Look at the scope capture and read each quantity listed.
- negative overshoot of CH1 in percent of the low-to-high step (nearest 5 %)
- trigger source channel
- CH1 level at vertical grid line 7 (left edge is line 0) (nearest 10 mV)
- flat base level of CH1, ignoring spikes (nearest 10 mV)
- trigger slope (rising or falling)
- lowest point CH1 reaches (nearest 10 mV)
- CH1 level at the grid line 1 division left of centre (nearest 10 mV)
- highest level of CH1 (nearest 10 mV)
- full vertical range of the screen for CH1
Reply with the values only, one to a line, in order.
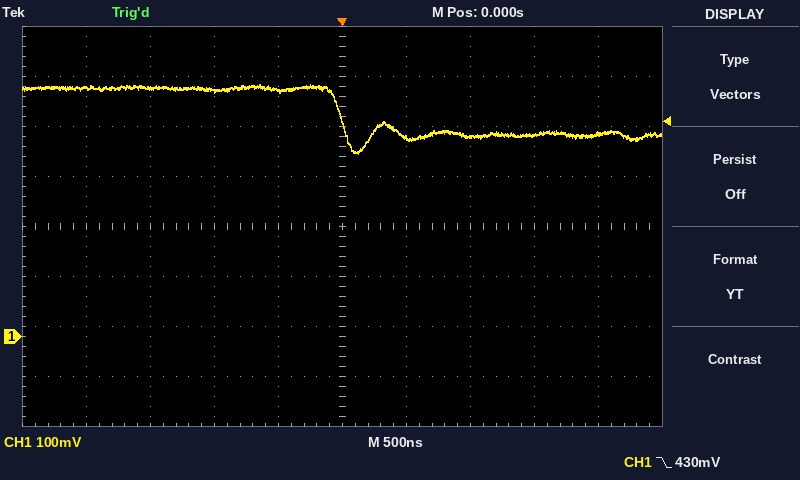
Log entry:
40 %
CH1
400 mV
400 mV
falling
370 mV
490 mV
500 mV
800 mV
